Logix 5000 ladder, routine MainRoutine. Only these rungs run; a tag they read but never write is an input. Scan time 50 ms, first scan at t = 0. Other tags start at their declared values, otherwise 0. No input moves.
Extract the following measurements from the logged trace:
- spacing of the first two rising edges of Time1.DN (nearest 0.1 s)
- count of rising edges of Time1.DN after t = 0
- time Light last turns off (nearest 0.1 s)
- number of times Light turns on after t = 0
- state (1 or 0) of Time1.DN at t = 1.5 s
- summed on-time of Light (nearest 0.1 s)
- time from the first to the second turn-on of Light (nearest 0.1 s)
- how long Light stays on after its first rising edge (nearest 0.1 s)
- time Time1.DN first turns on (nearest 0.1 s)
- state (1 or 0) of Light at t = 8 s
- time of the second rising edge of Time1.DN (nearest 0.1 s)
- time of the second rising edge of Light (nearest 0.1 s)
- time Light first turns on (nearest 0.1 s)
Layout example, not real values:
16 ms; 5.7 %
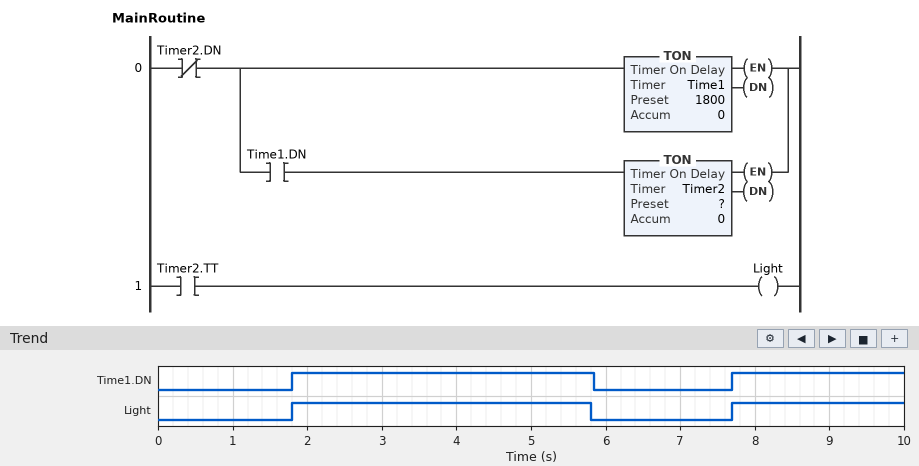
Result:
5.9 s; 2; 5.8 s; 2; 0; 6.3 s; 5.9 s; 4.0 s; 1.8 s; 1; 7.7 s; 7.7 s; 1.8 s
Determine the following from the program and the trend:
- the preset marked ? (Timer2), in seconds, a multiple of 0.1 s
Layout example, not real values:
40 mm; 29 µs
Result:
4.0 s
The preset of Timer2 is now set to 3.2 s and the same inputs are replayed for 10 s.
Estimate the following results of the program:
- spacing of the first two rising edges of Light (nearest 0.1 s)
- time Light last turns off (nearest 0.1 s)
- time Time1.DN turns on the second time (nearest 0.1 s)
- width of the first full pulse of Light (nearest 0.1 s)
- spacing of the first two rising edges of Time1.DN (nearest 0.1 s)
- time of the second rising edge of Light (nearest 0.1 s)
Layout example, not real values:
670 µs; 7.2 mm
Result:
5.1 s; 5.0 s; 6.9 s; 3.2 s; 5.1 s; 6.9 s
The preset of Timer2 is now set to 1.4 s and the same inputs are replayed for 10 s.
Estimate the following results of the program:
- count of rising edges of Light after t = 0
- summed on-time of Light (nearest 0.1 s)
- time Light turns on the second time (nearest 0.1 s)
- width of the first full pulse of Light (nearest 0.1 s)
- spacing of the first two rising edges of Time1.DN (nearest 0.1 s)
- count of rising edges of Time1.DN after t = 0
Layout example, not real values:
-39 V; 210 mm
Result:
3; 4.2 s; 5.1 s; 1.4 s; 3.3 s; 3
